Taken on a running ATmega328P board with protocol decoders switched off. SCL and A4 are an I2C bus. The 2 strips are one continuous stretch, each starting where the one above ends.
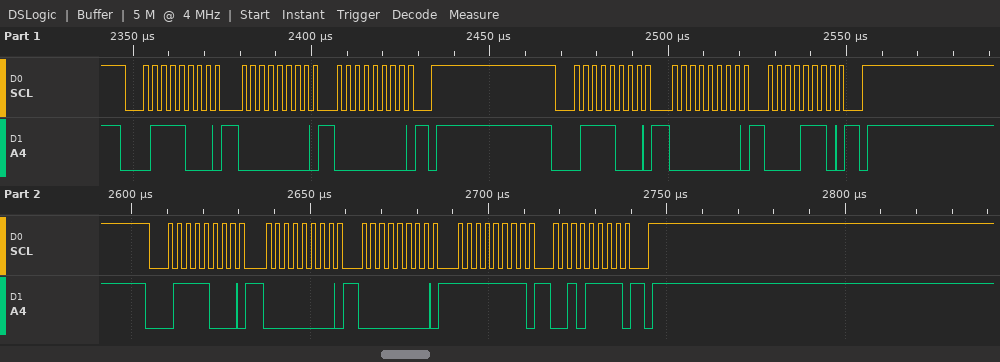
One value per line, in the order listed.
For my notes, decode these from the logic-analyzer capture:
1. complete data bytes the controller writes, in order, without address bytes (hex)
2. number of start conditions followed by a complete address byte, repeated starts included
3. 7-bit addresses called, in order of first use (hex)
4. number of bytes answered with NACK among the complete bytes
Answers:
00 00 00 0E 00 00 FF 2F
3
0x3C
0
